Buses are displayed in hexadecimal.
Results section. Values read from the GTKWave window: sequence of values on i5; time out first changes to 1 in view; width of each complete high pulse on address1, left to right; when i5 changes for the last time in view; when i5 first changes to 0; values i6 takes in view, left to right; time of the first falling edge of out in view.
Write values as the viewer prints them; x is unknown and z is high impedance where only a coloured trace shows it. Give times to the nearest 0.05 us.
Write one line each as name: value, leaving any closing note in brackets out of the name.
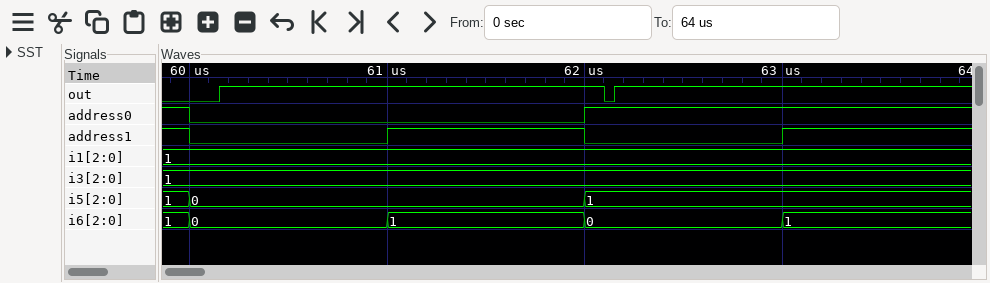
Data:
sequence of values on i5: 1, 0, 1
time out first changes to 1 in view: 60.15 us
width of each complete high pulse on address1, left to right: 1 us
when i5 changes for the last time in view: 62 us
when i5 first changes to 0: 60 us
values i6 takes in view, left to right: 1, 0, 1, 0, 1
time of the first falling edge of out in view: 62.1 us
